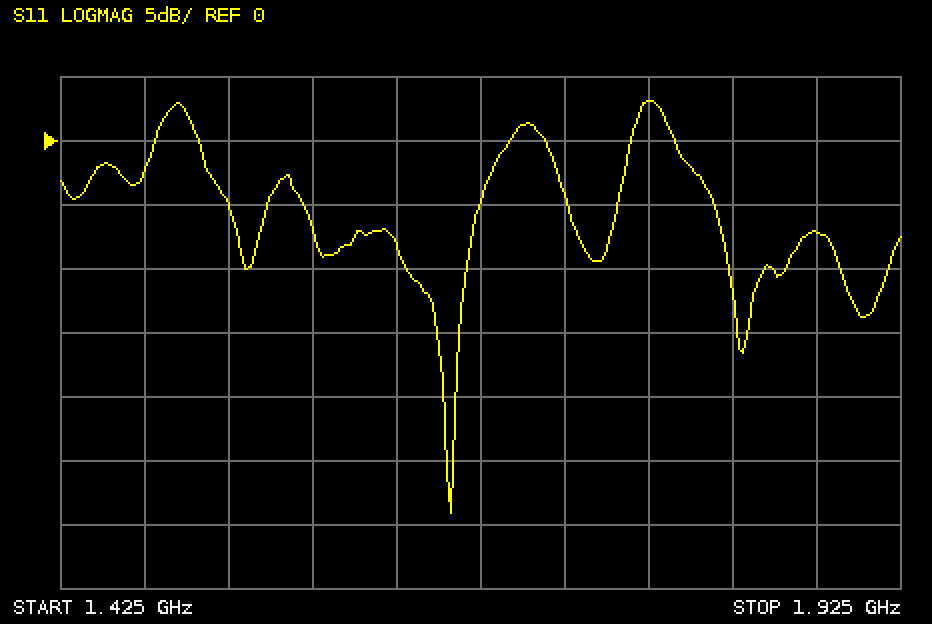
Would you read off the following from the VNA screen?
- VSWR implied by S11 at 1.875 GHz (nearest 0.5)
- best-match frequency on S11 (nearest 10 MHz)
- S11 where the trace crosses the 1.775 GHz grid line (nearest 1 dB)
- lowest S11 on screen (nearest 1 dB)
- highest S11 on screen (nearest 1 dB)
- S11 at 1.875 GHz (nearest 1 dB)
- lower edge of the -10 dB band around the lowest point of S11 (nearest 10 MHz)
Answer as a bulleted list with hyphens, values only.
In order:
- 2.5
- 1.66 GHz
- 3 dB
- -29 dB
- 3 dB
- -7 dB
- 1.63 GHz
